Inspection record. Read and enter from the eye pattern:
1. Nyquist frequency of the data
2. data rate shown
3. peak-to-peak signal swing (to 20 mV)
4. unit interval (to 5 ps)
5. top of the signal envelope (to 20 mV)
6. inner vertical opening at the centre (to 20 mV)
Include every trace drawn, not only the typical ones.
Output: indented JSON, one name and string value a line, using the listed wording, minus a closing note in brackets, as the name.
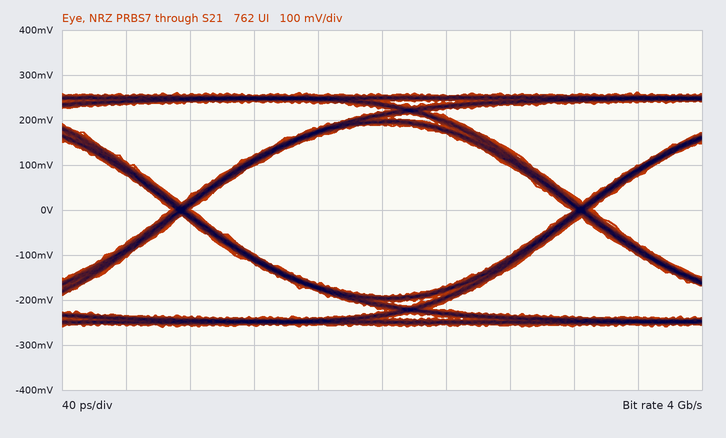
{
  "Nyquist frequency of the data": "2 GHz",
  "data rate shown": "4 Gb/s",
  "peak-to-peak signal swing": "520 mV",
  "unit interval": "250 ps",
  "top of the signal envelope": "260 mV",
  "inner vertical opening at the centre": "380 mV"
}
